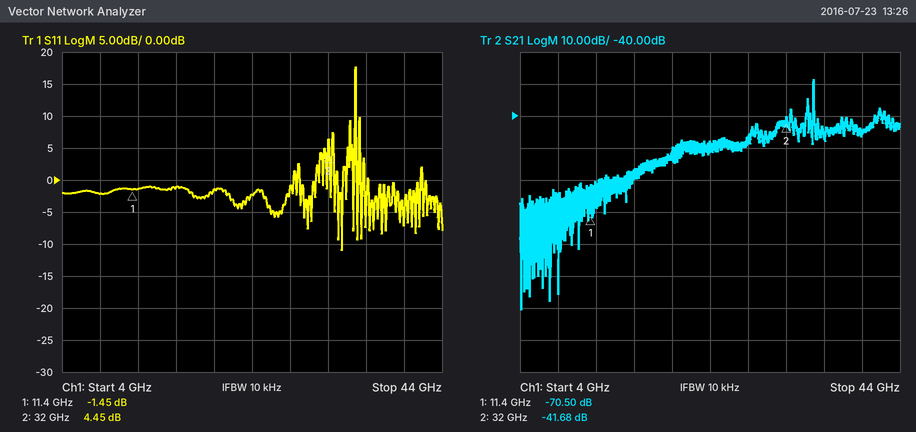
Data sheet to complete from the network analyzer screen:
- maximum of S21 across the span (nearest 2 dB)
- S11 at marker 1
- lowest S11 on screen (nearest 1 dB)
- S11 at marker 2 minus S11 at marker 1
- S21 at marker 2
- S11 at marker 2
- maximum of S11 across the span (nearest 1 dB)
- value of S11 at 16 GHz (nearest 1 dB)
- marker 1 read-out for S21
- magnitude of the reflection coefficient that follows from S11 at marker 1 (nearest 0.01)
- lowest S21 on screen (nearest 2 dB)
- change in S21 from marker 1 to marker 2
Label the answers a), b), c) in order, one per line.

a) -28 dB
b) -1.45 dB
c) -11 dB
d) 5.90 dB
e) -41.68 dB
f) 4.45 dB
g) 18 dB
h) -1 dB
i) -70.50 dB
j) 0.85
k) -100 dB
l) 28.82 dB
